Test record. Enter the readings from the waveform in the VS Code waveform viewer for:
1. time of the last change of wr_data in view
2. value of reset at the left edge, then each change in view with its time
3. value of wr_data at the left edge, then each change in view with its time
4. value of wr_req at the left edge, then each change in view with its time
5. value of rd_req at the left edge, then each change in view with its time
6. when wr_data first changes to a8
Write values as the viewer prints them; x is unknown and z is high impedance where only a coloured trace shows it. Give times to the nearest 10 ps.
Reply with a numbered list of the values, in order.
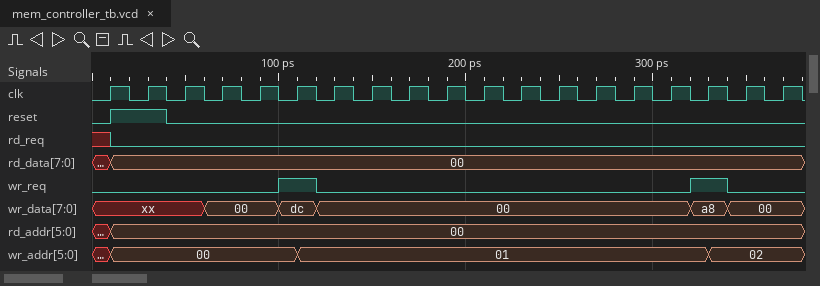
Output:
1. 340 ps
2. 0, 1 at 10 ps, 0 at 40 ps
3. xx, 00 at 60 ps, dc at 100 ps, 00 at 120 ps, a8 at 320 ps, 00 at 340 ps
4. 0, 1 at 100 ps, 0 at 120 ps, 1 at 320 ps, 0 at 340 ps
5. x, 0 at 10 ps
6. 320 ps
